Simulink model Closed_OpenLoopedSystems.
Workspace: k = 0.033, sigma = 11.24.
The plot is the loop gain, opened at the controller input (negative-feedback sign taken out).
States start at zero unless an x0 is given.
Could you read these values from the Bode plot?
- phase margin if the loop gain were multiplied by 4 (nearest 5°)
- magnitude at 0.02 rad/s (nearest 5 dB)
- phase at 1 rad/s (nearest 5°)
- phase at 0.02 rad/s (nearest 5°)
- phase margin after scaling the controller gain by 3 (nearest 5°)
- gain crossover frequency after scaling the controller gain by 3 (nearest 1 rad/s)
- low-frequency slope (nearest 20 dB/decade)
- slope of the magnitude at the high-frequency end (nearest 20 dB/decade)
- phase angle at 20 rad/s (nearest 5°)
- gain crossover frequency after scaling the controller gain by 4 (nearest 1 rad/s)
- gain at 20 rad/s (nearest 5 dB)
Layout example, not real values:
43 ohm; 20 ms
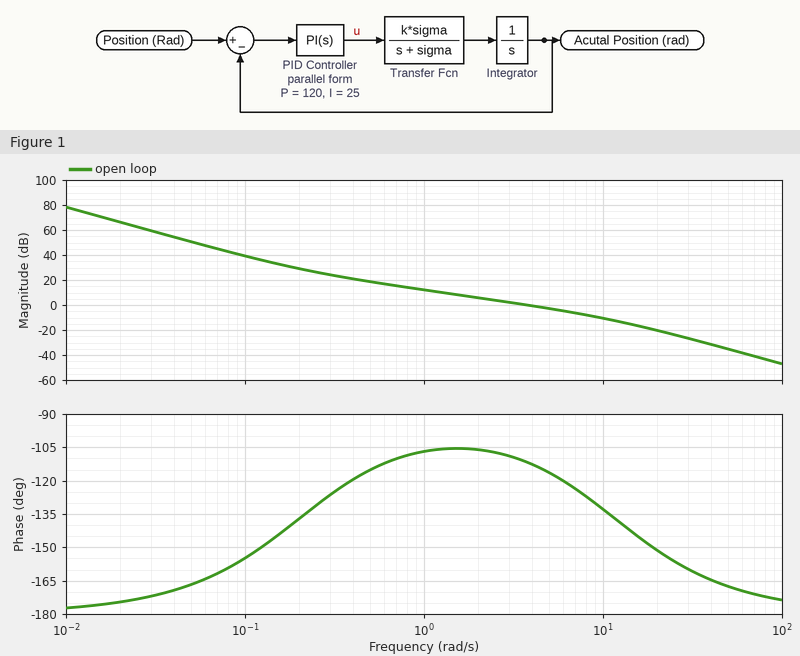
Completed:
45°; 65 dB; -105°; -175°; 50°; 9 rad/s; -40 dB/decade; -40 dB/decade; -150°; 11 rad/s; -20 dB
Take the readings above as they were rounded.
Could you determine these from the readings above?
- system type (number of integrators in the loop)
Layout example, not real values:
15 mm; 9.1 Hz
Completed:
2
